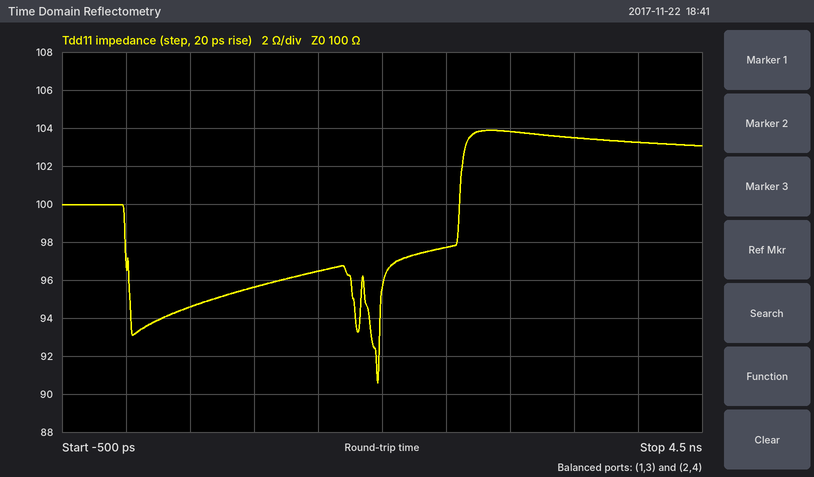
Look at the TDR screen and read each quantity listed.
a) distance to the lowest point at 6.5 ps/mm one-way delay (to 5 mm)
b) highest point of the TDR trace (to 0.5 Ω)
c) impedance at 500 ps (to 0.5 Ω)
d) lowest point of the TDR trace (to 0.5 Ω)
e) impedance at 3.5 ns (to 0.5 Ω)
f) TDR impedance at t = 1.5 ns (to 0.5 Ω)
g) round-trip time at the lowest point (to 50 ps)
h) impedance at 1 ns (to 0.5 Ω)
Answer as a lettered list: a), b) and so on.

a) 150 mm
b) 104.0 Ω
c) 94.5 Ω
d) 90.5 Ω
e) 103.5 Ω
f) 96.5 Ω
g) 1.95 ns
h) 95.5 Ω
